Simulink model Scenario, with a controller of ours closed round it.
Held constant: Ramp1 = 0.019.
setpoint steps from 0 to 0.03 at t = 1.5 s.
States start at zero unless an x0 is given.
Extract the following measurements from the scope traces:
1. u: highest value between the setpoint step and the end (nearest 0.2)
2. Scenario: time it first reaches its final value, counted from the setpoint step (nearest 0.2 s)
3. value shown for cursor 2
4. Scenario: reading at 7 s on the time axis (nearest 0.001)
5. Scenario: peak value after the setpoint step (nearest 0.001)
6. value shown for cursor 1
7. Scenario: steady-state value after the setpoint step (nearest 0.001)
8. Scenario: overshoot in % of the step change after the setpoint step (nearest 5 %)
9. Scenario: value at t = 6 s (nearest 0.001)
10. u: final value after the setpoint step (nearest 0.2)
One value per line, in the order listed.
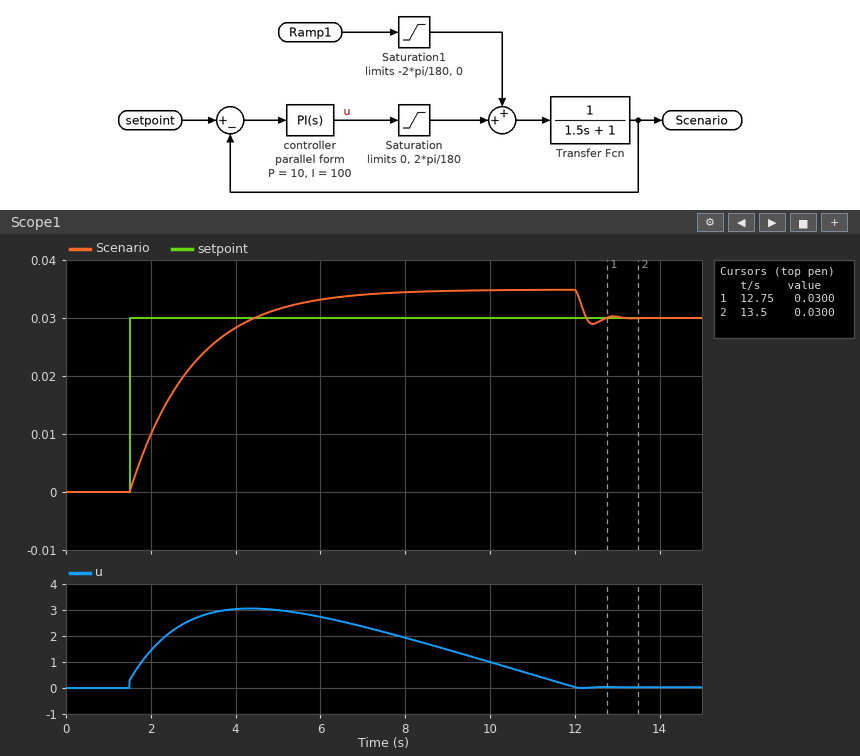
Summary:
3.0
3.0 s
0.0300
0.034
0.035
0.0300
0.030
15 %
0.033
0.0
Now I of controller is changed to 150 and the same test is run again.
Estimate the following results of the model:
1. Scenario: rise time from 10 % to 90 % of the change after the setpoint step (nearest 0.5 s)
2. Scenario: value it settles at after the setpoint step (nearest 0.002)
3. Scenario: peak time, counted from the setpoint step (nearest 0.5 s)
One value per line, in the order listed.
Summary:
2.0 s
0.030
10.5 s
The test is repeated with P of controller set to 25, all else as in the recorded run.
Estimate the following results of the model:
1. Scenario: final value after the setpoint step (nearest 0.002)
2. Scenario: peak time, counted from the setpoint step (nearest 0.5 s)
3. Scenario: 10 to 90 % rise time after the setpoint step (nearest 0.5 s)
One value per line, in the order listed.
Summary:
0.030
10.5 s
2.0 s
